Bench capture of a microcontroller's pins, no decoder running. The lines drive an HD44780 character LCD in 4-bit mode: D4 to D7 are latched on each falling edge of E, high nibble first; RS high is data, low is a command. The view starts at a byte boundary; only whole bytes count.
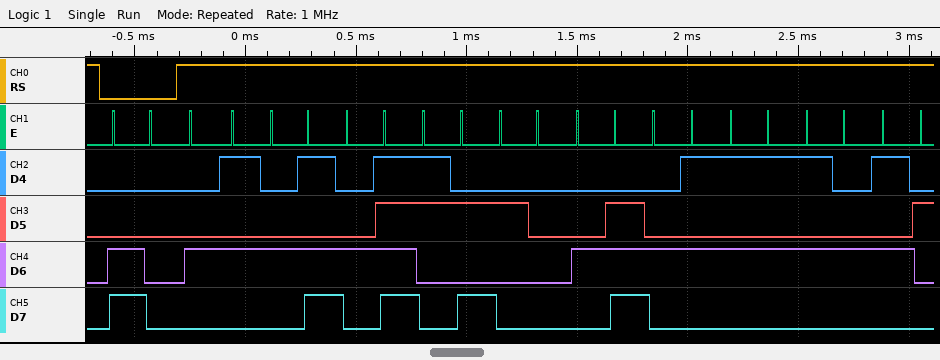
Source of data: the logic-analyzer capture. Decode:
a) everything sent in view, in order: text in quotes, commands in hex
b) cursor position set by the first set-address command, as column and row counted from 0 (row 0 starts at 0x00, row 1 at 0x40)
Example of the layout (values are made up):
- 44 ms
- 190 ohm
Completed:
- 0xC0 "EMO: NEUTR"
- column 0, row 1
